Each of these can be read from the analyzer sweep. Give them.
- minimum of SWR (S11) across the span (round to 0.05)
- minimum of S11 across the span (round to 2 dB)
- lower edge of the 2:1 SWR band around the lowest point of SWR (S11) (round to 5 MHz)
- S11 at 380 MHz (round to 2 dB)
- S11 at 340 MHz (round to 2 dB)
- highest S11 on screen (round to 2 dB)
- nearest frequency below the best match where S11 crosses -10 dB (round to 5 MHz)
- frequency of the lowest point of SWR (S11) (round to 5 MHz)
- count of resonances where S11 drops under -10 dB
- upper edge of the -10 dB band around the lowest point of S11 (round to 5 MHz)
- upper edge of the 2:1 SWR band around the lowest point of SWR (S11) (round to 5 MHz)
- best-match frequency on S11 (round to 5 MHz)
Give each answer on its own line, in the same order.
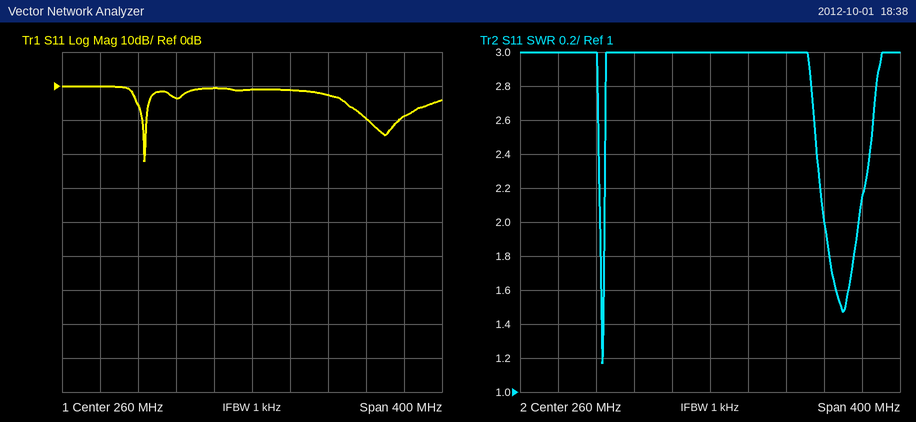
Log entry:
1.15
-22 dB
145 MHz
-10 dB
-2 dB
0 dB
145 MHz
145 MHz
2
150 MHz
150 MHz
145 MHz
